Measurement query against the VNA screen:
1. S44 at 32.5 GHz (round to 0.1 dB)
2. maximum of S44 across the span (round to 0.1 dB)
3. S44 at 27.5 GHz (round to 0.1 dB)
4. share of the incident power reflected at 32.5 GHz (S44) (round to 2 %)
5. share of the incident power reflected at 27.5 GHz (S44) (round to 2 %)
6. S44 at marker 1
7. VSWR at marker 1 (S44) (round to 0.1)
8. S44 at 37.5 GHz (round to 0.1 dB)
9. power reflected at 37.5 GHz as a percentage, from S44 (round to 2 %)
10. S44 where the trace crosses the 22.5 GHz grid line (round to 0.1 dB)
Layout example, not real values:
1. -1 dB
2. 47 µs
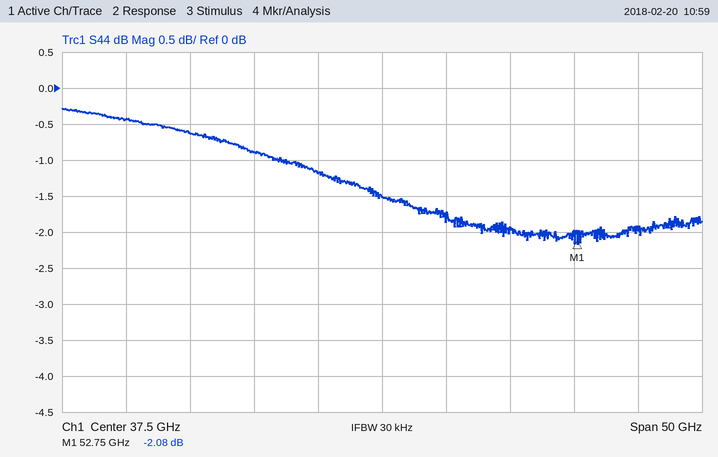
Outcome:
1. -1.2 dB
2. -0.3 dB
3. -0.9 dB
4. 76 %
5. 82 %
6. -2.08 dB
7. 8.4
8. -1.5 dB
9. 70 %
10. -0.6 dB
